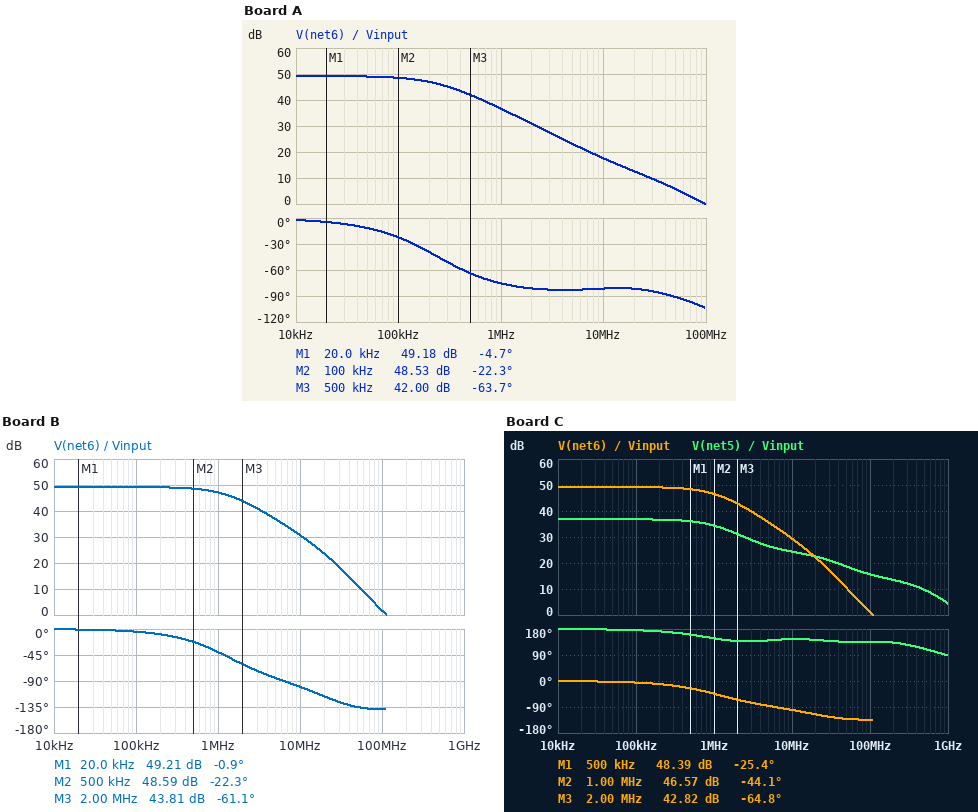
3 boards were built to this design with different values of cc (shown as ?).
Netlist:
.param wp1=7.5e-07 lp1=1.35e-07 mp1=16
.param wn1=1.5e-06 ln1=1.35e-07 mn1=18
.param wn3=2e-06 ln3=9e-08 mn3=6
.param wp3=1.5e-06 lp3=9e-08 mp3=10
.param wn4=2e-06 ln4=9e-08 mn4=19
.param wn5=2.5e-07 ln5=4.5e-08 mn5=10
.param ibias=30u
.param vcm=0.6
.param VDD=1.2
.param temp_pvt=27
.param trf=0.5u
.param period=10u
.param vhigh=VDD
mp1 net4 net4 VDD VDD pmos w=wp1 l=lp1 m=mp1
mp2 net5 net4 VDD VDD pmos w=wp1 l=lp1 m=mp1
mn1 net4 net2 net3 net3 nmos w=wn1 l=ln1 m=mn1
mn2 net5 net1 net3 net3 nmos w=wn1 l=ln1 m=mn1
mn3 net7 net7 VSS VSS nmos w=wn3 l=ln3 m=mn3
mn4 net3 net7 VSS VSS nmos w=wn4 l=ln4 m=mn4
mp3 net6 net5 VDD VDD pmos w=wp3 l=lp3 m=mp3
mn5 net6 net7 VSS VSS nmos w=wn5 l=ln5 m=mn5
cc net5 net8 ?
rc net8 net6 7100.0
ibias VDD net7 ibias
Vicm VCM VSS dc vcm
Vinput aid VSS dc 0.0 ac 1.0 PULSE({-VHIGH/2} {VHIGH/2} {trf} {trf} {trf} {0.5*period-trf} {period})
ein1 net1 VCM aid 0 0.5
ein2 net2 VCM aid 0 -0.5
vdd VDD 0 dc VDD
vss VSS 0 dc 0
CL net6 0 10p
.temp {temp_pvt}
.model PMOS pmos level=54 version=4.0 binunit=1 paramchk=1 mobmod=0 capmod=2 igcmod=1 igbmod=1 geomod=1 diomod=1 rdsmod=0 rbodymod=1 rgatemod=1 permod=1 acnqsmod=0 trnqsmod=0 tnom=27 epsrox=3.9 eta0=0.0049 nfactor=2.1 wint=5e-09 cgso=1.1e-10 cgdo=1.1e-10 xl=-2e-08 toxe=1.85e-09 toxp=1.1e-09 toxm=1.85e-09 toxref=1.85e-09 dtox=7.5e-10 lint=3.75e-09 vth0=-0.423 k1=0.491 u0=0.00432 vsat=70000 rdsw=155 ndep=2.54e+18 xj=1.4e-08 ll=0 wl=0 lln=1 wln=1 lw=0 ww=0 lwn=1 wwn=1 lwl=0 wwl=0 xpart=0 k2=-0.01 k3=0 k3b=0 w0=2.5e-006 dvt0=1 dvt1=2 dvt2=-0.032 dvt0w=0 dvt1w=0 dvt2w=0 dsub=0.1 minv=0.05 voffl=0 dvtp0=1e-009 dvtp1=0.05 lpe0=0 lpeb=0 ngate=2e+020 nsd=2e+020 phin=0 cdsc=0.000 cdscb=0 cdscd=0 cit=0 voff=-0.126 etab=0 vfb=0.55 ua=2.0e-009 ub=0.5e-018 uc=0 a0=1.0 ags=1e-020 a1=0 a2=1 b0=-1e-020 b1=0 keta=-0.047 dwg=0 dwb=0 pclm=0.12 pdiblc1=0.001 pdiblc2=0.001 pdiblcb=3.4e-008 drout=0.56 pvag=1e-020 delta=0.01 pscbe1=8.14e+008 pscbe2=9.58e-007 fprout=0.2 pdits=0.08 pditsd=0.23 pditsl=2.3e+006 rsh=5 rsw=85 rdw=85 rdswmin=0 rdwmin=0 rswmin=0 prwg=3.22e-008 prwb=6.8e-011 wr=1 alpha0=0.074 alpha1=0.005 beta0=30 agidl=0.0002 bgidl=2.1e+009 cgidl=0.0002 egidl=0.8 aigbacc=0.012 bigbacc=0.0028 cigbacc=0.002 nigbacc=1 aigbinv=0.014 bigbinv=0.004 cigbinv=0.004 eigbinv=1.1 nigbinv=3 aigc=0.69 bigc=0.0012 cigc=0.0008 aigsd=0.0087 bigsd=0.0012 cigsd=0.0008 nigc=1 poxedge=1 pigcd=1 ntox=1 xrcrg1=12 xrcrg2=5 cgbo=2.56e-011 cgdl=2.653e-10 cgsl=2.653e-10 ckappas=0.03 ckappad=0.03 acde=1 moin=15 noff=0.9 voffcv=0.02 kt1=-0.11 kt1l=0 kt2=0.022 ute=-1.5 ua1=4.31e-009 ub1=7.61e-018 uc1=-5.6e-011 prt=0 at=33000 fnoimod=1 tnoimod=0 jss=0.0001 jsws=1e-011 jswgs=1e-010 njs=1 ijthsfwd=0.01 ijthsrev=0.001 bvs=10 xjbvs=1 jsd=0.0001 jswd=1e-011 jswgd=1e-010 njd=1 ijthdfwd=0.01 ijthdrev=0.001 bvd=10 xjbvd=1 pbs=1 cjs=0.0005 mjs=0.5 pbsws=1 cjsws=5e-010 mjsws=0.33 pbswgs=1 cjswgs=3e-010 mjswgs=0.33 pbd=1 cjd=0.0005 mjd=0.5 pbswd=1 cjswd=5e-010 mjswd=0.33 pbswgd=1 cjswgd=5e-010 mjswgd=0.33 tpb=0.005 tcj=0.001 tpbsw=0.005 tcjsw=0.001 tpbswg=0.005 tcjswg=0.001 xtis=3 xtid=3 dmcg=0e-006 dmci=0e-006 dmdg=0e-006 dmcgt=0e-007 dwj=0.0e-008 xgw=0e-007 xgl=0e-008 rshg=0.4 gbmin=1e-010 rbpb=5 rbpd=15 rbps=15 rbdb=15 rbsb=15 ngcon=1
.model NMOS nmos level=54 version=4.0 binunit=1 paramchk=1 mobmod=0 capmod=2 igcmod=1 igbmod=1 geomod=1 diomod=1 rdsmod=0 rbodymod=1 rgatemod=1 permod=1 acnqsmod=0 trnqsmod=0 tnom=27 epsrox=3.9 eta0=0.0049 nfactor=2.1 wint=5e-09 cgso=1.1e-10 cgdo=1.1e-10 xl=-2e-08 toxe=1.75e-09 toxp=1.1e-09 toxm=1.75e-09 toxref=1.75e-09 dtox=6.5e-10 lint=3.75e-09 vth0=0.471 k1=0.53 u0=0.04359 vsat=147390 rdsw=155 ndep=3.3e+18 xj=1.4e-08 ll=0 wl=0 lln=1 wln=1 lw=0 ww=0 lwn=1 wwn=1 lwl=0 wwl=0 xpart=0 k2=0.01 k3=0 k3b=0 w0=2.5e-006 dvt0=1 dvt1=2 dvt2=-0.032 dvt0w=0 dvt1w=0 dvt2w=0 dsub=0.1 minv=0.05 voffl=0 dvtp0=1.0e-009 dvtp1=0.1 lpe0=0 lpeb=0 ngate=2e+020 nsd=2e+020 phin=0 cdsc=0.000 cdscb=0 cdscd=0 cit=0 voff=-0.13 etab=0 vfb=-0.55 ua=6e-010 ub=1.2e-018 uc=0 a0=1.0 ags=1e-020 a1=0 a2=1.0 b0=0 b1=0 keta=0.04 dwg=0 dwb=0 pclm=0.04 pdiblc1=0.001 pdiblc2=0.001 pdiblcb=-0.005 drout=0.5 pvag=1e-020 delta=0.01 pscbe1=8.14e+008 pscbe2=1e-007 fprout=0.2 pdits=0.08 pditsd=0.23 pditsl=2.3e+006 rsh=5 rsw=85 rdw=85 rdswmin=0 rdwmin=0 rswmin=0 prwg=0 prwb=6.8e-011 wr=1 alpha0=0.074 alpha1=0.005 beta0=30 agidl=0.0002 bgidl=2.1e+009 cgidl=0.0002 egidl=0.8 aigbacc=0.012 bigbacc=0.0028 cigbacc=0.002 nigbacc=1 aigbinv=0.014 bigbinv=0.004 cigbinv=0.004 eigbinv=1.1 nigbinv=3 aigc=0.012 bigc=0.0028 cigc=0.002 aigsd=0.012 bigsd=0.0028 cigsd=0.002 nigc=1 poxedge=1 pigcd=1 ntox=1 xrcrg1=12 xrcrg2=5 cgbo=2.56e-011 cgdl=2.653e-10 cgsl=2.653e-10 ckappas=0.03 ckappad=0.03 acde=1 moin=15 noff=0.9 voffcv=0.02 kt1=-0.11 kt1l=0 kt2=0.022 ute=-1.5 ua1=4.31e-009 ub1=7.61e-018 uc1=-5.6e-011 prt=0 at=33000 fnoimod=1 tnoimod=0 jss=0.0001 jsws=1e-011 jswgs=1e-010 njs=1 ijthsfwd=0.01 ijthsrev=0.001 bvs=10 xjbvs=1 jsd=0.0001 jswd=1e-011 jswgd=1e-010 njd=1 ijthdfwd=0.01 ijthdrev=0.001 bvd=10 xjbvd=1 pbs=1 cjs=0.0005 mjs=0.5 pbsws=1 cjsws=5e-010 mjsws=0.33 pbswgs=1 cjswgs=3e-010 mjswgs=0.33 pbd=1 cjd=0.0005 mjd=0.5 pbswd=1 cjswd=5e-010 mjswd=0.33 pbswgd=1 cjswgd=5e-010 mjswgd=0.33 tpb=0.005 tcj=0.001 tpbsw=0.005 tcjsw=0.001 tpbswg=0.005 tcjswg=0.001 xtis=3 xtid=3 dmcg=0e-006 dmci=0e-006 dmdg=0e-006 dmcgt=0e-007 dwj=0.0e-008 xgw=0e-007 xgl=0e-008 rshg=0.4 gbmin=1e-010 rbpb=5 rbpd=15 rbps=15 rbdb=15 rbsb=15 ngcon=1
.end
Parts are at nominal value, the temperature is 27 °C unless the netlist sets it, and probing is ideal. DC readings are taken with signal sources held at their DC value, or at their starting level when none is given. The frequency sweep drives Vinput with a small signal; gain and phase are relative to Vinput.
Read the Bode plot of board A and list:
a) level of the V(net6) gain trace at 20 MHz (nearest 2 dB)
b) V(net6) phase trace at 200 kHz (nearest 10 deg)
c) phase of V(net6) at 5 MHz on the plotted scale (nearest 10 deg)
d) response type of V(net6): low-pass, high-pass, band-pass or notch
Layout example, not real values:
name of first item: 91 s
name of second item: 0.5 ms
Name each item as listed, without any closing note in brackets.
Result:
level of the V(net6) gain trace at 20 MHz: 12 dB
V(net6) phase trace at 200 kHz: -40 deg
phase of V(net6) at 5 MHz on the plotted scale: -80 deg
response type of V(net6): low-pass, high-pass, band-pass or notch: low-pass
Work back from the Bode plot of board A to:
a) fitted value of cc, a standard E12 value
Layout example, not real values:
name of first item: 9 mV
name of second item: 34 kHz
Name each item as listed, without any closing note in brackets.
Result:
fitted value of cc, a standard E12 value: 1.5 pF
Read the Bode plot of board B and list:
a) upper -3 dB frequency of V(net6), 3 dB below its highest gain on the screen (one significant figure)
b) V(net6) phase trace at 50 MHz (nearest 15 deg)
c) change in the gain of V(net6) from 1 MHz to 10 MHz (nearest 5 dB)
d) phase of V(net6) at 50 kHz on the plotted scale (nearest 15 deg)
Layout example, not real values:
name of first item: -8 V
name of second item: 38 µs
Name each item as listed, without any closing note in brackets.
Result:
upper -3 dB frequency of V(net6), 3 dB below its highest gain on the screen: 1 MHz
V(net6) phase trace at 50 MHz: -135 deg
change in the gain of V(net6) from 1 MHz to 10 MHz: -15 dB
phase of V(net6) at 50 kHz on the plotted scale: 0 deg
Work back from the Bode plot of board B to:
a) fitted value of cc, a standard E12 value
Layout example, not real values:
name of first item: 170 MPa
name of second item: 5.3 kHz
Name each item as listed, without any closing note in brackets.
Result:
fitted value of cc, a standard E12 value: 220 fF
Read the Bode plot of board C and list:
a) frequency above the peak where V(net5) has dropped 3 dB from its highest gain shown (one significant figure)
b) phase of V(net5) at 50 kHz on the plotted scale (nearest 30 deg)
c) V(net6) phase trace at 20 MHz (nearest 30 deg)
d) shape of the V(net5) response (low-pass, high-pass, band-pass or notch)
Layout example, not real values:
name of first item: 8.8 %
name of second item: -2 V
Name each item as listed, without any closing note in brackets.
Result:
frequency above the peak where V(net5) has dropped 3 dB from its highest gain shown: 1 MHz
phase of V(net5) at 50 kHz on the plotted scale: 180 deg
V(net6) phase trace at 20 MHz: -120 deg
shape of the V(net5) response: low-pass
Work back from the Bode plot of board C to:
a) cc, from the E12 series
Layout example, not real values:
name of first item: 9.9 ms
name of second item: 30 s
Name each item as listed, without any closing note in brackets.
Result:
cc, from the E12 series: 270 fF
